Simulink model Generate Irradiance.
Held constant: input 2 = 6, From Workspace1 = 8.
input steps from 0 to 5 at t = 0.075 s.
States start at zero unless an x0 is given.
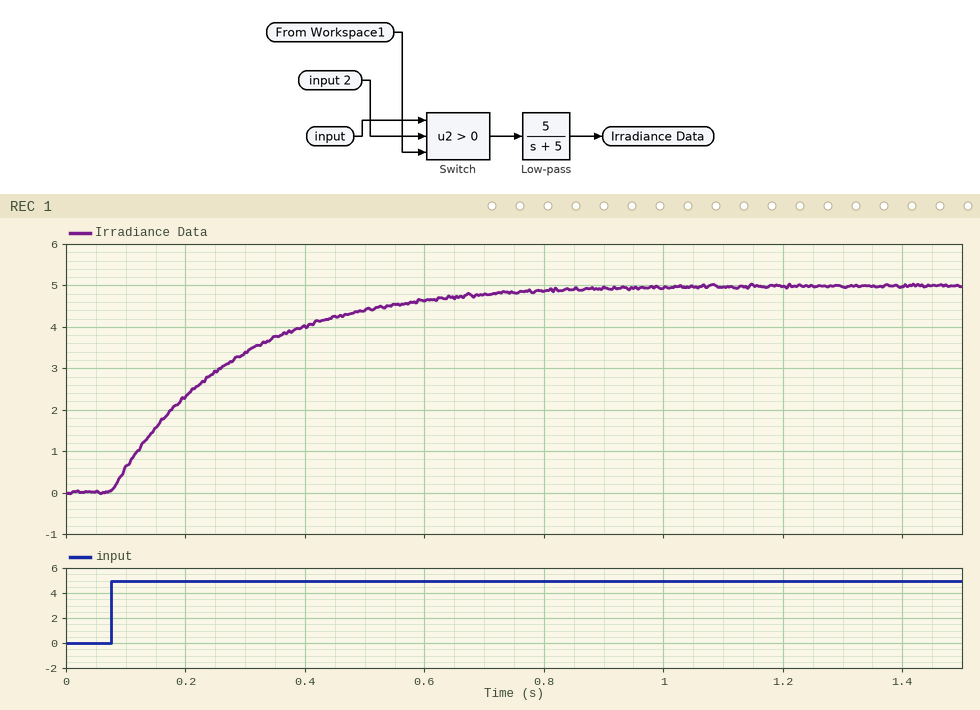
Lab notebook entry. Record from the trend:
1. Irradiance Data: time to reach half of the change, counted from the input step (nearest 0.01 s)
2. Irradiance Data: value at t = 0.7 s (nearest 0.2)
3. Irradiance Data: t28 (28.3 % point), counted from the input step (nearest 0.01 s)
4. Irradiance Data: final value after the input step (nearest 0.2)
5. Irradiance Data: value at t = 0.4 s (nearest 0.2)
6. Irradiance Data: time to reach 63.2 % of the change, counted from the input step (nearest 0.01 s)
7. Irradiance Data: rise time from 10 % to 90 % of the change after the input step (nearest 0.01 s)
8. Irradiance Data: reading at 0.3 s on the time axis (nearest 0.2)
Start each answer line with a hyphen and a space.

- 0.14 s
- 4.8
- 0.07 s
- 5.0
- 4.0
- 0.20 s
- 0.44 s
- 3.4
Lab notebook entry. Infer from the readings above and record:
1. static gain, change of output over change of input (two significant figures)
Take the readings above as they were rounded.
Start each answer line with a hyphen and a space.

- 1.0
